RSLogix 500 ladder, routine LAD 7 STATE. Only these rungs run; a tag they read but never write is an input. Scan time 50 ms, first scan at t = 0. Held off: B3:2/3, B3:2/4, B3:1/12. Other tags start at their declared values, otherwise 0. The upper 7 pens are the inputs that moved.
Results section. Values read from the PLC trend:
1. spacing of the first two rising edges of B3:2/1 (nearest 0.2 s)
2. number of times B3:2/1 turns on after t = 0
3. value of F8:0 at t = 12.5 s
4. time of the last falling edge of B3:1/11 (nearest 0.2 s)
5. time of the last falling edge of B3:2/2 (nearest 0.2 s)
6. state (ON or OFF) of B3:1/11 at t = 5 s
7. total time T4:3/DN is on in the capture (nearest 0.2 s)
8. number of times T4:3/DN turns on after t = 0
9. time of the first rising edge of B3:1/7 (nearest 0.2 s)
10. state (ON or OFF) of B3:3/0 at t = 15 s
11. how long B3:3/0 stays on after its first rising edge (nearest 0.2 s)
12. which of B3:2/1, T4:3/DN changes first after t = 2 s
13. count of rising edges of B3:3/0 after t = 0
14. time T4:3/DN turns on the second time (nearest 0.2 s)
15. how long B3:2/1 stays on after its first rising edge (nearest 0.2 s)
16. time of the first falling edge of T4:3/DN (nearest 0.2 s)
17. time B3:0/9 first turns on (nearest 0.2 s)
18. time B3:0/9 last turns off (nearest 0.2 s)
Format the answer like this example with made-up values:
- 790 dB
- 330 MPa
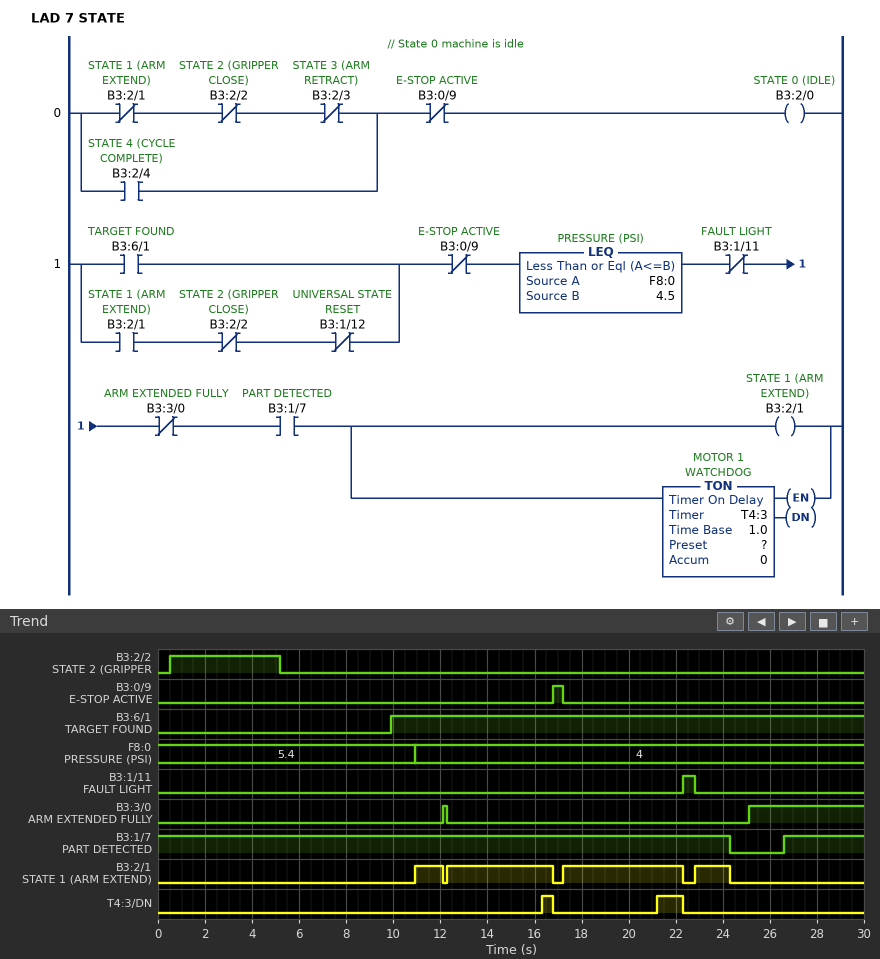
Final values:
- 1.4 s
- 4
- 4
- 22.8 s
- 5.2 s
- OFF
- 1.6 s
- 2
- 26.6 s
- OFF
- 0.2 s
- B3:2/1
- 2
- 21.2 s
- 1.2 s
- 16.8 s
- 16.8 s
- 17.2 s
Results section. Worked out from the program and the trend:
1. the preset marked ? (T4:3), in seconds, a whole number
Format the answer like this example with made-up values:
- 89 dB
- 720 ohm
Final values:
- 4 s
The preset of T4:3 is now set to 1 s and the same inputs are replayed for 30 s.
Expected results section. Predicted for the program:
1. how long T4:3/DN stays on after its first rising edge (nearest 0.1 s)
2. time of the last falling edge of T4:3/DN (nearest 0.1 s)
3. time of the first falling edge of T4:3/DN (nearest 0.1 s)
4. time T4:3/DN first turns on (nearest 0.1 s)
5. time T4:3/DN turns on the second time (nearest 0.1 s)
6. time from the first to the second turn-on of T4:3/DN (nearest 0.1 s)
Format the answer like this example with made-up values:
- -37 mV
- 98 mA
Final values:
- 0.2 s
- 24.3 s
- 12.1 s
- 11.9 s
- 13.3 s
- 1.4 s
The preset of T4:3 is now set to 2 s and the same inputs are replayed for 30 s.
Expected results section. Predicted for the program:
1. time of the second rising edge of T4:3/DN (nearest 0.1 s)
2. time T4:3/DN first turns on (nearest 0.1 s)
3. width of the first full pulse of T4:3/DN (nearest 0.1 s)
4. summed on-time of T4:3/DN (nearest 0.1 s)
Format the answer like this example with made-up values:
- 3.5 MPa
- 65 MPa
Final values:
- 19.2 s
- 14.3 s
- 2.5 s
- 5.6 s
